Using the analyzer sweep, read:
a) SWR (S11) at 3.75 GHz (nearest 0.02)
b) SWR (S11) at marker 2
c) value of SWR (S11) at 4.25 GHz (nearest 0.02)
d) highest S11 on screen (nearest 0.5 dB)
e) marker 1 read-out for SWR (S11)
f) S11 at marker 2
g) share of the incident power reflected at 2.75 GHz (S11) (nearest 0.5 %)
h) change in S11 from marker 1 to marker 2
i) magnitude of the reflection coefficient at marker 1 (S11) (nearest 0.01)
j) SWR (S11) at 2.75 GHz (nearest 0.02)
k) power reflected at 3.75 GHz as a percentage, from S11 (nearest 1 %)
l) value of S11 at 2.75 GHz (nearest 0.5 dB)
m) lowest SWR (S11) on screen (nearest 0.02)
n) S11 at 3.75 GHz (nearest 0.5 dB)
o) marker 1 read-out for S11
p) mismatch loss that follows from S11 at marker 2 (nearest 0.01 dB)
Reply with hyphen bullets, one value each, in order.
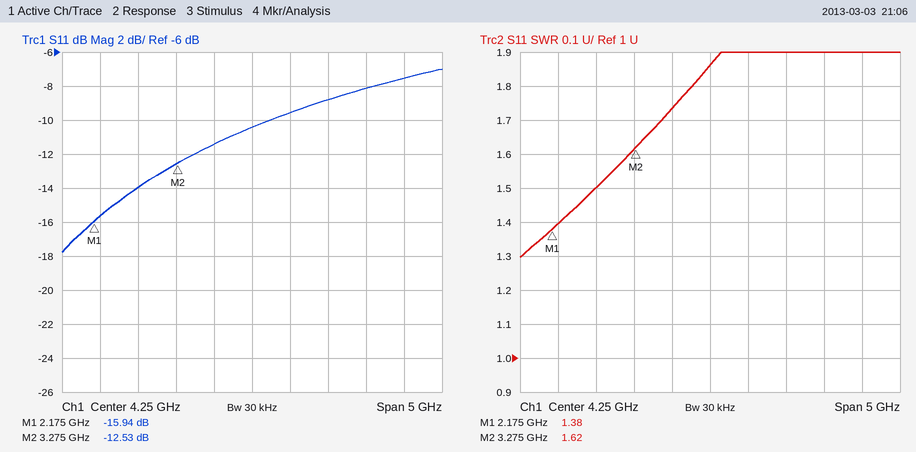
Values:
- 1.74
- 1.62
- 1.86
- -7.0 dB
- 1.38
- -12.53 dB
- 4.0 %
- 3.41 dB
- 0.16
- 1.50
- 7 %
- -14.0 dB
- 1.30
- -11.5 dB
- -15.94 dB
- 0.25 dB
